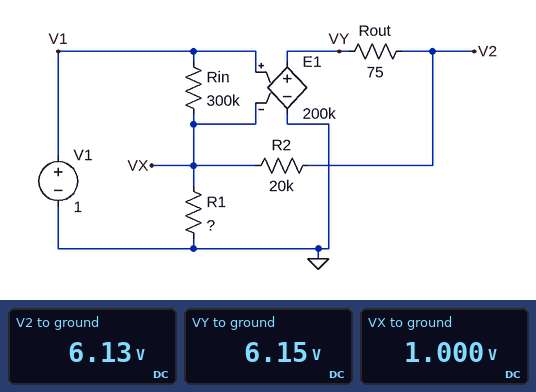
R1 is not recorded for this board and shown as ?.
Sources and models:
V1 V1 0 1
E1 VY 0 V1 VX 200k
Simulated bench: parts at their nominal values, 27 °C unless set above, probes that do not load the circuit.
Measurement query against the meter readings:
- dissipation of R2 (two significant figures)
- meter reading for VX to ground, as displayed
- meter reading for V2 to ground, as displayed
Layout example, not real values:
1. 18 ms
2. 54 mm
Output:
1. 1.3 mW
2. 1.000 V
3. 6.13 V
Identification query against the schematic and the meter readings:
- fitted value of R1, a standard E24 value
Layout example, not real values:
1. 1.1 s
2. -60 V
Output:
1. 3.9 kΩ
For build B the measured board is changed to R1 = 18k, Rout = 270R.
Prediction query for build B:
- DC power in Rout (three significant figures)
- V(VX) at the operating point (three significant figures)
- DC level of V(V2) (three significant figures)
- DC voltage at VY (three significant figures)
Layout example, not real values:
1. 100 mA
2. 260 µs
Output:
1. 833 nW
2. 1.00 V
3. 2.11 V
4. 2.13 V
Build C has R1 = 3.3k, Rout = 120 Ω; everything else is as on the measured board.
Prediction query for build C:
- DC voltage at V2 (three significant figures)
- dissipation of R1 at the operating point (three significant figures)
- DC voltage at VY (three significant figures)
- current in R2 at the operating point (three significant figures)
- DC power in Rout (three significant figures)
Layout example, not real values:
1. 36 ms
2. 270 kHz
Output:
1. 7.06 V
2. 303 µW
3. 7.10 V
4. 303 µA
5. 11.0 µW
